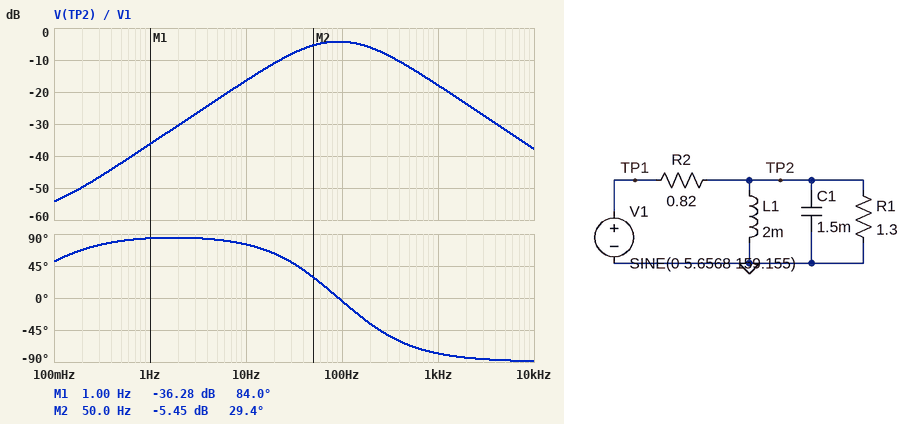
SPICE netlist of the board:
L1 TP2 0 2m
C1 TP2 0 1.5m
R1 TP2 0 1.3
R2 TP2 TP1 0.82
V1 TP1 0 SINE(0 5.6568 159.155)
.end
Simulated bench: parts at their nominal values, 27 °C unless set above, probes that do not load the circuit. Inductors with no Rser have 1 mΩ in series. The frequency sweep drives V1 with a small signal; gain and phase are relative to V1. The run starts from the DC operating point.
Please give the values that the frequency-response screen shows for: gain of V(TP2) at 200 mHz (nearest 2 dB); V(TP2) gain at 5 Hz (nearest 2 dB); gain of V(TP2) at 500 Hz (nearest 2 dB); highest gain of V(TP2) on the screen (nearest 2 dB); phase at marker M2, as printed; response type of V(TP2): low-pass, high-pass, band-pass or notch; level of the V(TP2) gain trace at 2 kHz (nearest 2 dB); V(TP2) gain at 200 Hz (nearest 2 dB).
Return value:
-50 dB
-22 dB
-12 dB
-4 dB
29.4 deg
band-pass
-24 dB
-6 dB
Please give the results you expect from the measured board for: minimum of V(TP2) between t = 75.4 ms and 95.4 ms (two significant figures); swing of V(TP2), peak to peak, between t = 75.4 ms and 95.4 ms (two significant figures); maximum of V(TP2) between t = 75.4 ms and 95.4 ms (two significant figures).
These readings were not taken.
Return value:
-3.1 V
6.2 V
3.1 V
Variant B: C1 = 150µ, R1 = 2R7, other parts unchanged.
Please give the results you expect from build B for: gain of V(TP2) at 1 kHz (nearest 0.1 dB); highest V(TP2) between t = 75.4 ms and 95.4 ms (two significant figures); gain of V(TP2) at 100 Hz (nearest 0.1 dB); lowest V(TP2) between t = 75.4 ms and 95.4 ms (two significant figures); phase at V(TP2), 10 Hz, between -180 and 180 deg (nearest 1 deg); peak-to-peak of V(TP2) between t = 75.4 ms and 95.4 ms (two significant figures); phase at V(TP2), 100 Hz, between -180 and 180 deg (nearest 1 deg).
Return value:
-3.4 dB
4.2 V
-3.1 dB
-4.2 V
78 deg
8.5 V
24 deg
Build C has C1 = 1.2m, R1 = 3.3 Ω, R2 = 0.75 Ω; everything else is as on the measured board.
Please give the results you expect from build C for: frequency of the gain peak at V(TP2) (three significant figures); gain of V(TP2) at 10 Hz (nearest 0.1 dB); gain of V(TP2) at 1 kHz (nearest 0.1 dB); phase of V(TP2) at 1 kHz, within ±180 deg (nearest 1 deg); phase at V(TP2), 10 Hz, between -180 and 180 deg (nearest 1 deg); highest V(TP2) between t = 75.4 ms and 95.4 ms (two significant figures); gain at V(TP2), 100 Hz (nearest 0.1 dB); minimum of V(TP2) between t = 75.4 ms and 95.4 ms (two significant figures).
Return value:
103 Hz
-15.6 dB
-15.2 dB
-78 deg
78 deg
4.2 V
-1.8 dB
-4.2 V
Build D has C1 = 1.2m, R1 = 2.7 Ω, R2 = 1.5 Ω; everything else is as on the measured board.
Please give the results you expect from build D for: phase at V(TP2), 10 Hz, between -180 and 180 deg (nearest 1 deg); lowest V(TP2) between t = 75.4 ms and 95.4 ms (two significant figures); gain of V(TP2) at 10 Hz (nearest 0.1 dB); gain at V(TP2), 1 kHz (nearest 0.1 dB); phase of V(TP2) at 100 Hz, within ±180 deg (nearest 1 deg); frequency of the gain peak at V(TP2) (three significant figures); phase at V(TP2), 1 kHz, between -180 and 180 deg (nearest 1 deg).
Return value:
82 deg
-3.0 V
-21.5 dB
-21.1 dB
2 deg
103 Hz
-82 deg
